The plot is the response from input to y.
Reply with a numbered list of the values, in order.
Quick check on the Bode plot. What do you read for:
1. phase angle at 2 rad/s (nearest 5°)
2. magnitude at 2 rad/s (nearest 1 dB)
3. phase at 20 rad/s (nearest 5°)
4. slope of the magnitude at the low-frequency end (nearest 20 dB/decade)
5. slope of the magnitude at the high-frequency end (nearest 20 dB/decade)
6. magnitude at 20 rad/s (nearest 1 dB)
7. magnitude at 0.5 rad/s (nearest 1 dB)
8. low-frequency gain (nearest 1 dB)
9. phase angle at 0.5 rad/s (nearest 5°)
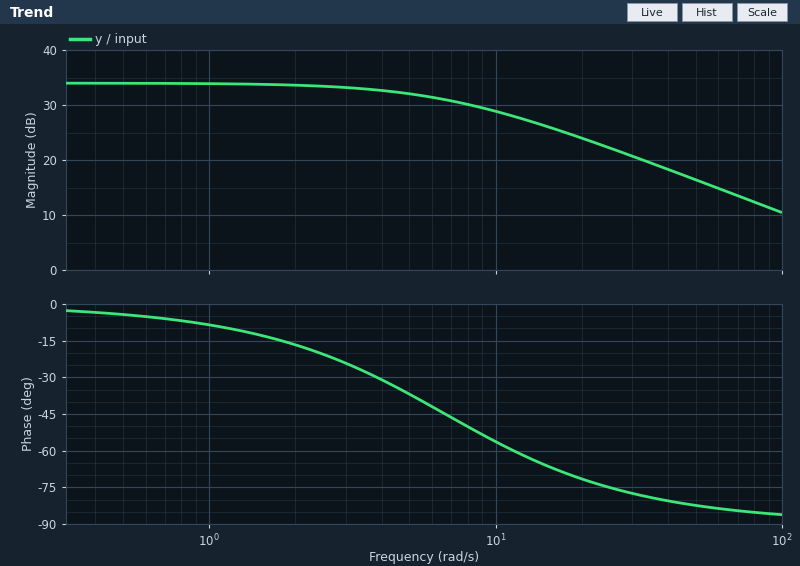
1. -15°
2. 34 dB
3. -70°
4. 0 dB/decade
5. -20 dB/decade
6. 24 dB
7. 34 dB
8. 34 dB
9. -5°
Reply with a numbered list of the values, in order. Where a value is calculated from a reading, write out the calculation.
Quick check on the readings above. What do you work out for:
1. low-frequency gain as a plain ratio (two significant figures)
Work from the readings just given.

1. 10^(34 / 20) = 50
